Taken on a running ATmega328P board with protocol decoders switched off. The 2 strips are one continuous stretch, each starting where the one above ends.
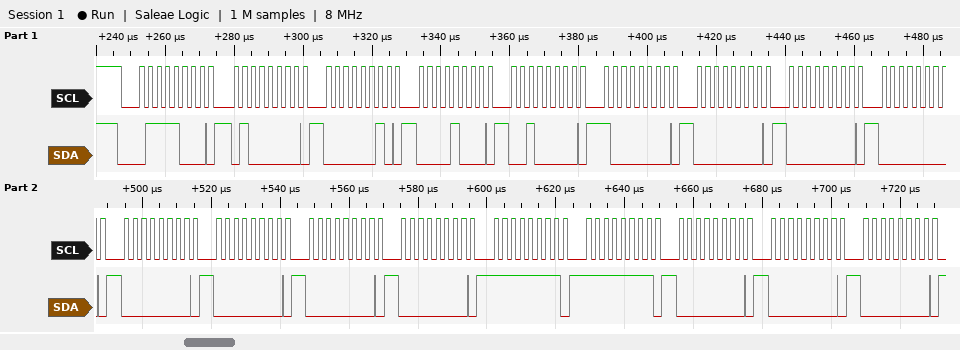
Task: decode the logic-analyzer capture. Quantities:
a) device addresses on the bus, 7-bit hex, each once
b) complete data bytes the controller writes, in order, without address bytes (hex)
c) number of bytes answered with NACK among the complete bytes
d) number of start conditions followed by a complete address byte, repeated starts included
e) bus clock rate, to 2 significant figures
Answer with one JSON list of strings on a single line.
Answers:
["0x3C", "40 02 08 20 80 00 00 00 00 00 00 00 FF FF 00 00 00", "0", "1", "400 kHz"]
